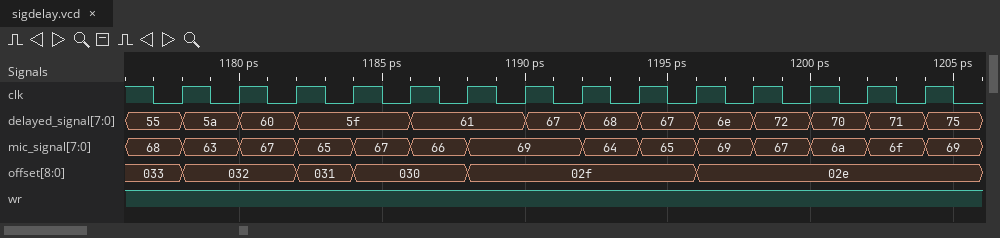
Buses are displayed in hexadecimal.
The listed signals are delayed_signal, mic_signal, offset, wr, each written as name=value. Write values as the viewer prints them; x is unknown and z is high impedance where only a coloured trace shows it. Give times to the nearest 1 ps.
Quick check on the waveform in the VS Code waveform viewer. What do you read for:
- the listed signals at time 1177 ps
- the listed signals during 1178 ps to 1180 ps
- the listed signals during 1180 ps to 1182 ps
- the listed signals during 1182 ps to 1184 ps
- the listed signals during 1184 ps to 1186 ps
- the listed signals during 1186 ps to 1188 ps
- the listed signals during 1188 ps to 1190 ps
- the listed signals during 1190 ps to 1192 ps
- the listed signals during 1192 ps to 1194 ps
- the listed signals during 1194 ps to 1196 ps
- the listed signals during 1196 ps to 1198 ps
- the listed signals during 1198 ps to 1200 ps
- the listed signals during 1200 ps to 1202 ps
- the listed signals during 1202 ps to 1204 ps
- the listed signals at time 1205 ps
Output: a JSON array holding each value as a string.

["delayed_signal=55, mic_signal=68, offset=033, wr=1", "delayed_signal=5a, mic_signal=63, offset=032, wr=1", "delayed_signal=60, mic_signal=67, offset=032, wr=1", "delayed_signal=5f, mic_signal=65, offset=031, wr=1", "delayed_signal=5f, mic_signal=67, offset=030, wr=1", "delayed_signal=61, mic_signal=66, offset=030, wr=1", "delayed_signal=61, mic_signal=69, offset=02f, wr=1", "delayed_signal=67, mic_signal=69, offset=02f, wr=1", "delayed_signal=68, mic_signal=64, offset=02f, wr=1", "delayed_signal=67, mic_signal=65, offset=02f, wr=1", "delayed_signal=6e, mic_signal=69, offset=02e, wr=1", "delayed_signal=72, mic_signal=67, offset=02e, wr=1", "delayed_signal=70, mic_signal=6a, offset=02e, wr=1", "delayed_signal=71, mic_signal=6f, offset=02e, wr=1", "delayed_signal=75, mic_signal=69, offset=02e, wr=1"]
